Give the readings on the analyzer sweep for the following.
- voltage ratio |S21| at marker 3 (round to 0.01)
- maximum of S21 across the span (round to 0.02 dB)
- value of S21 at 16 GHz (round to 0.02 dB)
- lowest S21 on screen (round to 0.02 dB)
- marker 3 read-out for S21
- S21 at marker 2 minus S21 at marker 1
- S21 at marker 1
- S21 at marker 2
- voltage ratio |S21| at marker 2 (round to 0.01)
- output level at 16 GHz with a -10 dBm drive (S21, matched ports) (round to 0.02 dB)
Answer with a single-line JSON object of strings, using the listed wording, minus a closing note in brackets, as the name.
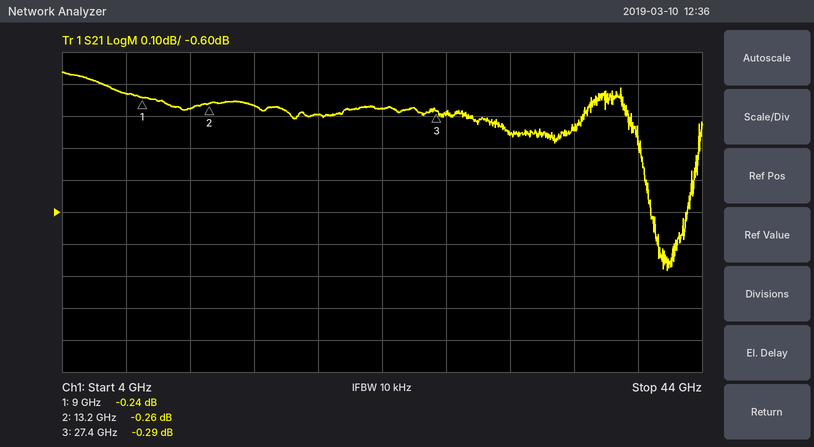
{"voltage ratio |S21| at marker 3": "0.97", "maximum of S21 across the span": "-0.16 dB", "value of S21 at 16 GHz": "-0.26 dB", "lowest S21 on screen": "-0.78 dB", "marker 3 read-out for S21": "-0.29 dB", "S21 at marker 2 minus S21 at marker 1": "-0.02 dB", "S21 at marker 1": "-0.24 dB", "S21 at marker 2": "-0.26 dB", "voltage ratio |S21| at marker 2": "0.97", "output level at 16 GHz with a -10 dBm drive (S21, matched ports)": "-10.26 dBm"}
